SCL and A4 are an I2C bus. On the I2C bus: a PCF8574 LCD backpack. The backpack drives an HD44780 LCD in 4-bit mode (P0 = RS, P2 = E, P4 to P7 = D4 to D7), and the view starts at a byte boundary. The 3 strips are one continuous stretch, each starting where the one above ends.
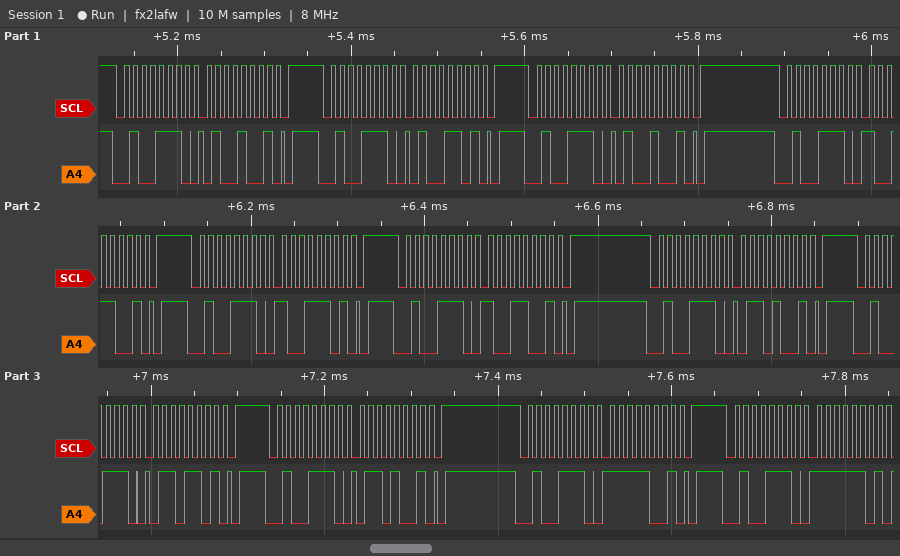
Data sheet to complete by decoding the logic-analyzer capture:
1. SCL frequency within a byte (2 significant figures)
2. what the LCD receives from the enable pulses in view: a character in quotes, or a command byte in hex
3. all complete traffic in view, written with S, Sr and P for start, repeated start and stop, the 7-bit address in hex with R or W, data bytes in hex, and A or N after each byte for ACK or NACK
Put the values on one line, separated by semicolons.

100 kHz; 'I'; S 27W A 49 A P S 27W A 4D A P S 27W A 49 A P S 27W A 99 A P S 27W A 9D A P S 27W A 99 A P S 27W A 69 A P S 27W A 6D A P S 27W A 69 A P S 27W A F9 A P S 27W A FD A
